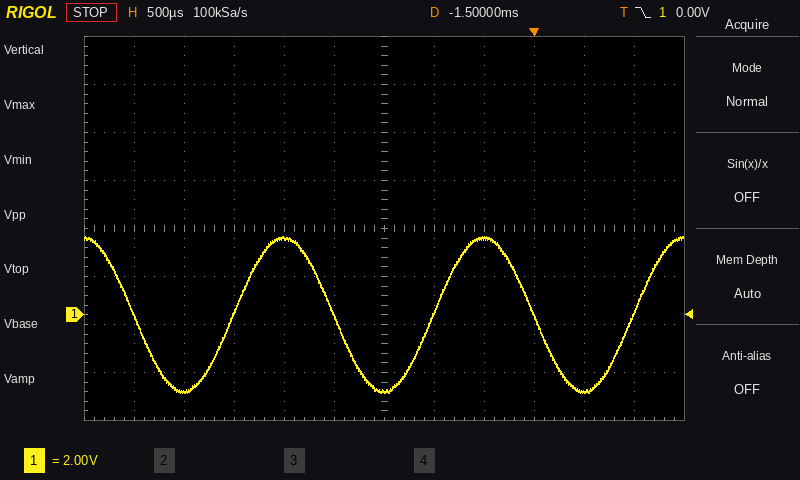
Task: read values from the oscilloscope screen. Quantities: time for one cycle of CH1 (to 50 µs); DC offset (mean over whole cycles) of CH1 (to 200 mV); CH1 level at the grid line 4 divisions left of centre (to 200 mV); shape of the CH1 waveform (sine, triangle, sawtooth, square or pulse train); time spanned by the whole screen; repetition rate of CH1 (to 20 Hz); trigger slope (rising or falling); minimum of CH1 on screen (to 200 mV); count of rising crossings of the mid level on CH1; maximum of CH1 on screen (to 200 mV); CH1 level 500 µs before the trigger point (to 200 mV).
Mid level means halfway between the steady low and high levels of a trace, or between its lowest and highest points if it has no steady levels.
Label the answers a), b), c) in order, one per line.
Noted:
a) 2.00 ms
b) 0.0 V
c) -3.2 V
d) sine
e) 6 ms
f) 500 Hz
g) falling
h) -3.2 V
i) 3
j) 3.2 V
k) 3.2 V
